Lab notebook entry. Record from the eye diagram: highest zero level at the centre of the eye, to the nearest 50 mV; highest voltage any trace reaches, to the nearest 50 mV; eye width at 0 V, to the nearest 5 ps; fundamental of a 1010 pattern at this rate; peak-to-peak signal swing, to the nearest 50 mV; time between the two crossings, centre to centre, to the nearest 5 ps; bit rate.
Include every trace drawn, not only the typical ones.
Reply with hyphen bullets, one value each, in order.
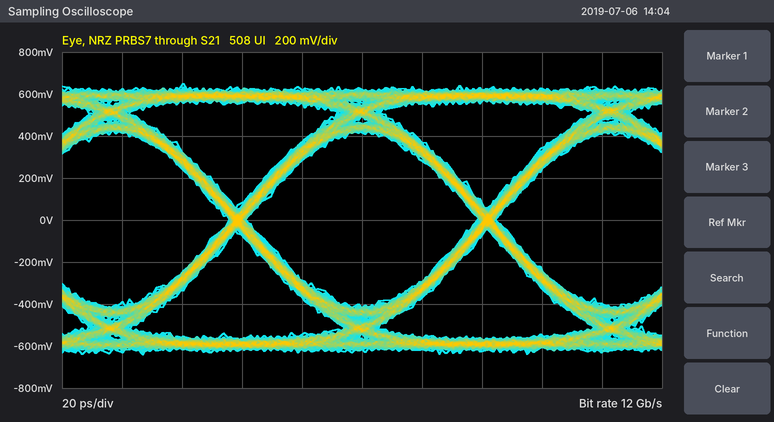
- -400 mV
- 650 mV
- 75 ps
- 6 GHz
- 1.30 V
- 85 ps
- 12 Gb/s
